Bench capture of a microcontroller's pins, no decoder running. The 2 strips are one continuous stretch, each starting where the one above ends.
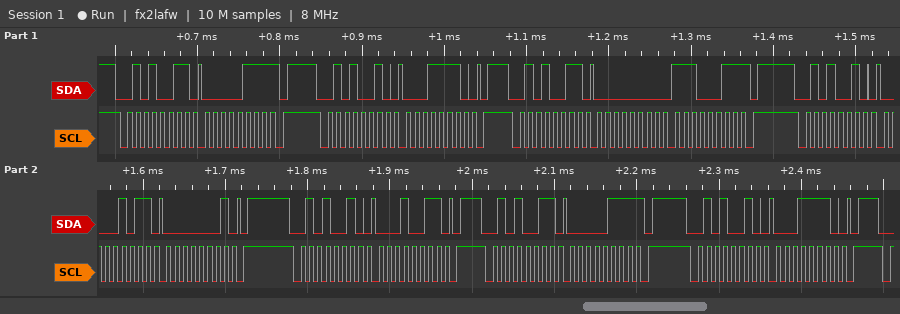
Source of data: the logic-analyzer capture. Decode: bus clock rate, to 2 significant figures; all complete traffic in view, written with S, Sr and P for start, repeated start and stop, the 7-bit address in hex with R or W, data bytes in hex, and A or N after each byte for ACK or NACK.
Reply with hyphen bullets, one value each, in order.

- 100 kHz
- S 29R A 07 N P S 29W A 1E A P S 29R A 00 A E3 N P S 29W A 0B A 01 A P S 29W A 13 A P S 29R A 07 N P S 29W A 1E A P
